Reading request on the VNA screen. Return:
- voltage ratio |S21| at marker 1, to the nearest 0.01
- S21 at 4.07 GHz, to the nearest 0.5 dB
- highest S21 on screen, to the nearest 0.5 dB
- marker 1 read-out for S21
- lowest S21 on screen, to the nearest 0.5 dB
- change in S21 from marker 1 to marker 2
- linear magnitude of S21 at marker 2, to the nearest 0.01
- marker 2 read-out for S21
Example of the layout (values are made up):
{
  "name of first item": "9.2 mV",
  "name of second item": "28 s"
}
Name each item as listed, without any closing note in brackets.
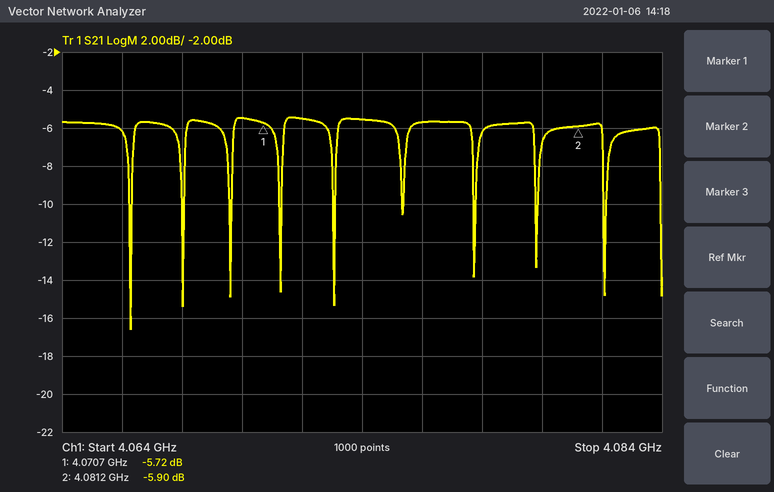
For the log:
{
  "voltage ratio |S21| at marker 1, to the nearest 0.01": "0.52",
  "S21 at 4.07 GHz, to the nearest 0.5 dB": "-5.5 dB",
  "highest S21 on screen, to the nearest 0.5 dB": "-5.5 dB",
  "marker 1 read-out for S21": "-5.72 dB",
  "lowest S21 on screen, to the nearest 0.5 dB": "-16.5 dB",
  "change in S21 from marker 1 to marker 2": "-0.18 dB",
  "linear magnitude of S21 at marker 2, to the nearest 0.01": "0.51",
  "marker 2 read-out for S21": "-5.90 dB"
}
